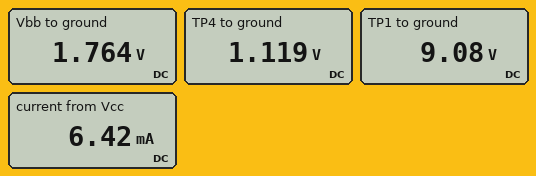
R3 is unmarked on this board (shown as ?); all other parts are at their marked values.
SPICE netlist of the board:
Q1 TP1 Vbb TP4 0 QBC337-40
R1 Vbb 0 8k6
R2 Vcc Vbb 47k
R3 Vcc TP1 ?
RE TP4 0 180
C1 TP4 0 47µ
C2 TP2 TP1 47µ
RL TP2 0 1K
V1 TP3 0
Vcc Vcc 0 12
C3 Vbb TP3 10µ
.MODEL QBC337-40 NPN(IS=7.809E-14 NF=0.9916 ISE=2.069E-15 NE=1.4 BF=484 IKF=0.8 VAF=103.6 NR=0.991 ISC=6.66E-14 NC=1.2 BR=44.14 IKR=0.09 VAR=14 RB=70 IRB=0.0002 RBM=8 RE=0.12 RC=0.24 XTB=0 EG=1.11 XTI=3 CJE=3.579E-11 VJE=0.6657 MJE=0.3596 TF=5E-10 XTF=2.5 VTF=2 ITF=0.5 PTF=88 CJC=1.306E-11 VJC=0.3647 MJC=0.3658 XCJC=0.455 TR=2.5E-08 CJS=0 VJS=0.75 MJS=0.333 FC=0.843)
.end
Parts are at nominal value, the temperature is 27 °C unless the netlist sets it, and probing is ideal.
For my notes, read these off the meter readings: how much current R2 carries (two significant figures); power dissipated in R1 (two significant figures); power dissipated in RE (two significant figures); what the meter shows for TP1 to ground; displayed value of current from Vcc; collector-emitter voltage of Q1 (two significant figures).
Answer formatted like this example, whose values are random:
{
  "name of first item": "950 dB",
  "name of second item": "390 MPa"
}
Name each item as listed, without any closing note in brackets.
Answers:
{
  "how much current R2 carries": "220 µA",
  "power dissipated in R1": "360 µW",
  "power dissipated in RE": "7.0 mW",
  "what the meter shows for TP1 to ground": "9.08 V",
  "displayed value of current from Vcc": "6.42 mA",
  "collector-emitter voltage of Q1": "8.0 V"
}
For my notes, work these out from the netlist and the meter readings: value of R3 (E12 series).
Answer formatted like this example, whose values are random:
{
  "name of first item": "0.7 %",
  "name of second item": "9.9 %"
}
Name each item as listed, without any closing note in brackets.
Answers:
{
  "value of R3": "470 Ω"
}
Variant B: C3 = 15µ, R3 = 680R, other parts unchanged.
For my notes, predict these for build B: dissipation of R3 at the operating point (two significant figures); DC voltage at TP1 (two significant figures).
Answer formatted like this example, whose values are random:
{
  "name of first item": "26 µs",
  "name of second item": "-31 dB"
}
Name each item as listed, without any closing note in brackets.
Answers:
{
  "dissipation of R3 at the operating point": "26 mW",
  "DC voltage at TP1": "7.8 V"
}
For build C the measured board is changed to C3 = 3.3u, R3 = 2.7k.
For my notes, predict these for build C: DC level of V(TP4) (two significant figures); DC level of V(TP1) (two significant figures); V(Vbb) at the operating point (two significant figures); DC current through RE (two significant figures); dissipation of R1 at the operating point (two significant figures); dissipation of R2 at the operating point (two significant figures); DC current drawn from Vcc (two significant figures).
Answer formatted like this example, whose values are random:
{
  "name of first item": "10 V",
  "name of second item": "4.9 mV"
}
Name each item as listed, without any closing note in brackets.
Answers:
{
  "DC level of V(TP4)": "760 mV",
  "DC level of V(TP1)": "800 mV",
  "V(Vbb) at the operating point": "1.4 V",
  "DC current through RE": "4.2 mA",
  "dissipation of R1 at the operating point": "230 µW",
  "dissipation of R2 at the operating point": "2.4 mW",
  "DC current drawn from Vcc": "4.4 mA"
}
